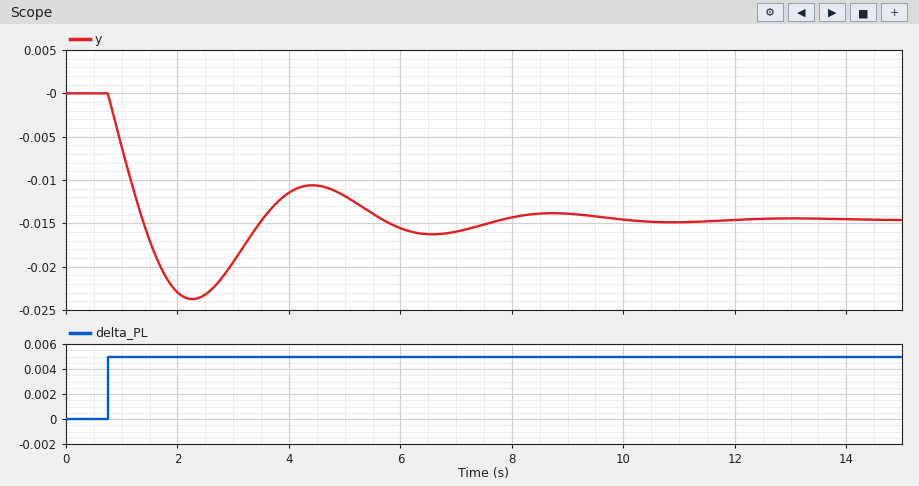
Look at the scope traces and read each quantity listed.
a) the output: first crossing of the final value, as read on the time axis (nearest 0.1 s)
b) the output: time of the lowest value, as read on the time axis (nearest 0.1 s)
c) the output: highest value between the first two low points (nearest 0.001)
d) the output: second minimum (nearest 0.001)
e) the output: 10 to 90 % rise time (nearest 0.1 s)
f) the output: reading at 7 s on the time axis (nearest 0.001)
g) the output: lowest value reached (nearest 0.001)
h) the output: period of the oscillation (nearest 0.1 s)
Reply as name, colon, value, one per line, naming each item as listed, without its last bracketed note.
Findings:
the output: first crossing of the final value, as read on the time axis: 1.4 s
the output: time of the lowest value, as read on the time axis: 2.3 s
the output: highest value between the first two low points: -0.011
the output: second minimum: -0.016
the output: 10 to 90 % rise time: 0.5 s
the output: reading at 7 s on the time axis: -0.016
the output: lowest value reached: -0.024
the output: period of the oscillation: 4.3 s
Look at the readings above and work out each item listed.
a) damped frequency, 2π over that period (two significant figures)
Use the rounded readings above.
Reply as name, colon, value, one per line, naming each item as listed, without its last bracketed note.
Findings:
damped frequency, 2π over that period: 1.5 rad/s
